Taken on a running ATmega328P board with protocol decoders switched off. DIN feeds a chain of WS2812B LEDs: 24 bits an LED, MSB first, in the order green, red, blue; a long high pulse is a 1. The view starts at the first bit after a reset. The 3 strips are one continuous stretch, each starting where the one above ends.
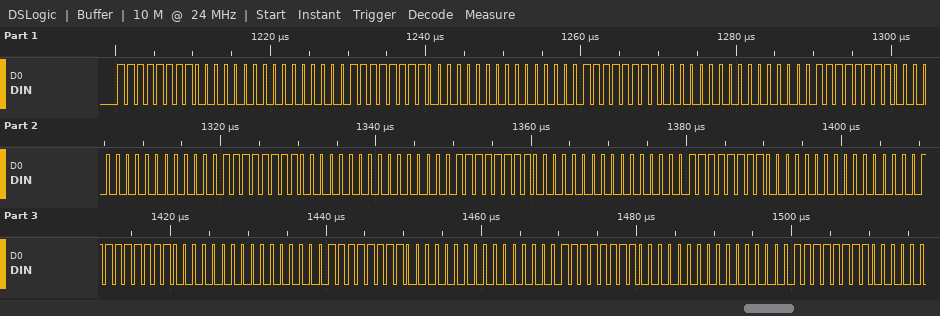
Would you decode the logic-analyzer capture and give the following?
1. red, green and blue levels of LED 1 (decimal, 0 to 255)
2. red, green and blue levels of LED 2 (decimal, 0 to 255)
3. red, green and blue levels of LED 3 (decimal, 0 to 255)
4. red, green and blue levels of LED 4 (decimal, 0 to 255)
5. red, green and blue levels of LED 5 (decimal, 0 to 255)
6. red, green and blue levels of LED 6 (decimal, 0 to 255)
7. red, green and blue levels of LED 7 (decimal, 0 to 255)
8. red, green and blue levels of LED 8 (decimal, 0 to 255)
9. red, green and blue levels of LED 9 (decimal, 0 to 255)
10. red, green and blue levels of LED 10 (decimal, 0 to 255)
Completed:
0, 255, 0
0, 255, 0
0, 255, 0
0, 255, 0
0, 255, 0
0, 255, 0
0, 255, 0
0, 255, 0
0, 255, 0
0, 255, 0
